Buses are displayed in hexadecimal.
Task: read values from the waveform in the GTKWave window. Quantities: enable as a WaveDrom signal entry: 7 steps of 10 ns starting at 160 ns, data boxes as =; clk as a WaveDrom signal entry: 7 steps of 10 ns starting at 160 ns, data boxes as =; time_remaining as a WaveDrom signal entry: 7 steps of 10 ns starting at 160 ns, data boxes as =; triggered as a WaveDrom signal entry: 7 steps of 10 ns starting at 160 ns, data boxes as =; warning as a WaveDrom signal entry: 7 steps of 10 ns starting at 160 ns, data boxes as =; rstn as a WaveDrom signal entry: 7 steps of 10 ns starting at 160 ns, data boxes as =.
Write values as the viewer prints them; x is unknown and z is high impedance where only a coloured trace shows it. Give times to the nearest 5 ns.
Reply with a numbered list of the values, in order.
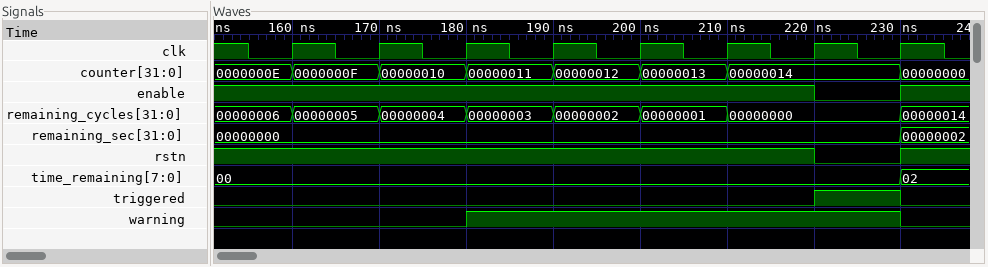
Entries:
1. {name: 'enable', wave: '1.....0'}
2. {name: 'clk', wave: 'p......'}
3. {name: 'time_remaining', wave: '=......', data: '00'}
4. {name: 'triggered', wave: '0.....1'}
5. {name: 'warning', wave: '0.1....'}
6. {name: 'rstn', wave: '1.....0'}
